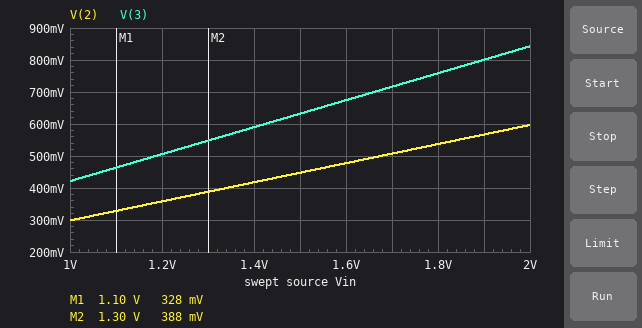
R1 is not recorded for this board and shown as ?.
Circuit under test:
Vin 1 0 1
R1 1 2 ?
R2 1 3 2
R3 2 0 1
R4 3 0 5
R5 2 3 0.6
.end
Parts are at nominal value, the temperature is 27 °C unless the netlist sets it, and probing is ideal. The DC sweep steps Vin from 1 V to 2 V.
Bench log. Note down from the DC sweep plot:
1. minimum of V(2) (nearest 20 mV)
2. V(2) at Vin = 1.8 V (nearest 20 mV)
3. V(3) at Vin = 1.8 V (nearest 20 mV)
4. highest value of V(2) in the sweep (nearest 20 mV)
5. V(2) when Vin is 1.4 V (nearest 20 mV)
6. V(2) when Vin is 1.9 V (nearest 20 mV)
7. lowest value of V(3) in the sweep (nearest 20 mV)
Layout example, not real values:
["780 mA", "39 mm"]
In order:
["300 mV", "540 mV", "760 mV", "600 mV", "420 mV", "560 mV", "420 mV"]
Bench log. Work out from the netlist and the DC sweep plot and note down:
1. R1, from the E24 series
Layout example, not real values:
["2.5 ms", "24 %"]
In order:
["7.5 Ω"]
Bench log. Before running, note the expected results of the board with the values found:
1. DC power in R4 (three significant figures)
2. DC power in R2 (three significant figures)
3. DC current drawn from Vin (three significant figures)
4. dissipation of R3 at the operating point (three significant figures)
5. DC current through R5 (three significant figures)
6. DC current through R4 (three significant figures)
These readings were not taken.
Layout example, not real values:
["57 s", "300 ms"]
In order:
["35.5 mW", "167 mW", "383 mA", "89.1 mW", "205 mA", "84.3 mA"]
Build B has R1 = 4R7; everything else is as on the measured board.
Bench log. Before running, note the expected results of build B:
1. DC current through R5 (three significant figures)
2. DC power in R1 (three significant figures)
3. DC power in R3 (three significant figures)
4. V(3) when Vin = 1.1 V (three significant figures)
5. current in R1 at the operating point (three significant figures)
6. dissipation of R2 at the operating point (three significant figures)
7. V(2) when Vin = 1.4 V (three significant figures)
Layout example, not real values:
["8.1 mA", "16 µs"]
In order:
["189 mA", "95.2 mW", "110 mW", "489 mV", "142 mA", "154 mW", "464 mV"]
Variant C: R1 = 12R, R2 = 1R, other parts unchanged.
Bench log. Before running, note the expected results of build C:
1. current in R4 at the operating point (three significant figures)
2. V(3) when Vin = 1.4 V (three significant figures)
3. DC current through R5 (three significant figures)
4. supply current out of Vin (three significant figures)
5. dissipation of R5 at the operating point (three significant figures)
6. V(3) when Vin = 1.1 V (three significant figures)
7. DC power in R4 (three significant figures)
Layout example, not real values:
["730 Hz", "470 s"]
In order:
["113 mA", "792 mV", "321 mA", "486 mA", "61.8 mW", "622 mV", "64.0 mW"]
